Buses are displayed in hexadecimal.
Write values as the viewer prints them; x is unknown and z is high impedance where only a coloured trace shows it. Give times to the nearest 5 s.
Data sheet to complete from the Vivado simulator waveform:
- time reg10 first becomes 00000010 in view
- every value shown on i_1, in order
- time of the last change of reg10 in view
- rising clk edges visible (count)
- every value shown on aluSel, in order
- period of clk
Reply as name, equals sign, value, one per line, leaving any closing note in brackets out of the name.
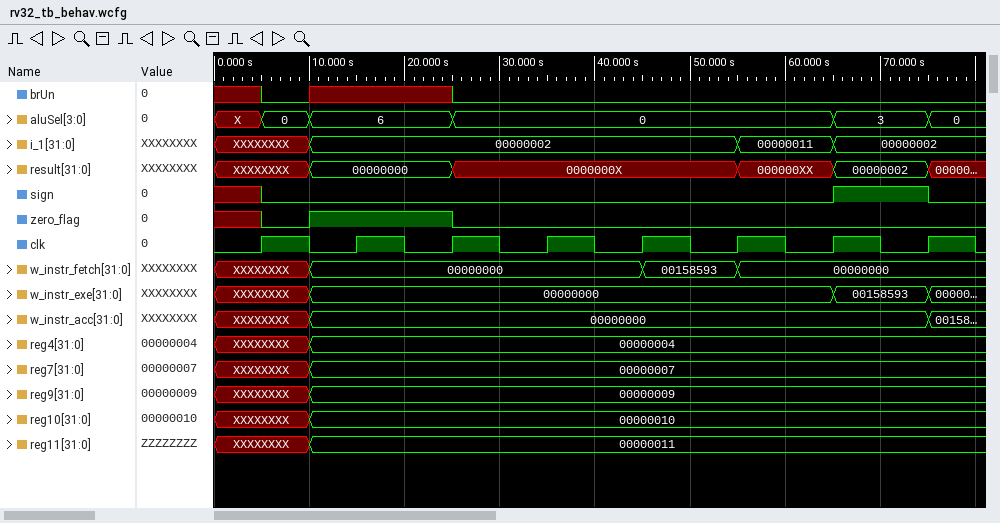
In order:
time reg10 first becomes 00000010 in view = 10 s
every value shown on i_1, in order = XXXXXXXX, 00000002, 00000011, 00000002
time of the last change of reg10 in view = 10 s
rising clk edges visible = 8
every value shown on aluSel, in order = X, 0, 6, 0, 3, 0
period of clk = 10 s
